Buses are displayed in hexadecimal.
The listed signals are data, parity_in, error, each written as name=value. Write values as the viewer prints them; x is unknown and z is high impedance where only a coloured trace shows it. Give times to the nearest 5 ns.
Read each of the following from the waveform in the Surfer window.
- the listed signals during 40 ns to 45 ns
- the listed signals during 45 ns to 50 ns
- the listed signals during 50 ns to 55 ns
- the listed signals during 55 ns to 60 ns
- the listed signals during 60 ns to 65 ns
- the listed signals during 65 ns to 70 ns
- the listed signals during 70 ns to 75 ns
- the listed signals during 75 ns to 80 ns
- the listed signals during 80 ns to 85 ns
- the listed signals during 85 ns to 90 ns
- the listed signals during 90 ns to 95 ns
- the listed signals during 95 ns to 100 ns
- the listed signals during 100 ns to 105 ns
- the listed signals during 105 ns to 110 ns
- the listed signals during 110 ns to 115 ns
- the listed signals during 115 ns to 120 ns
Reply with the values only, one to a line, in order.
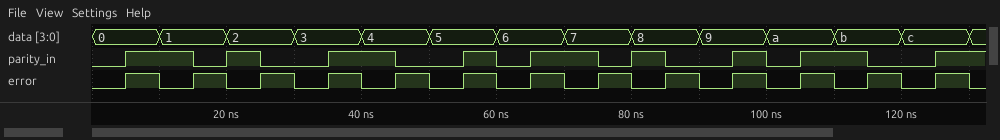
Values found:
data=4, parity_in=1, error=0
data=4, parity_in=0, error=1
data=5, parity_in=0, error=0
data=5, parity_in=1, error=1
data=6, parity_in=0, error=0
data=6, parity_in=1, error=1
data=7, parity_in=1, error=0
data=7, parity_in=0, error=1
data=8, parity_in=1, error=0
data=8, parity_in=0, error=1
data=9, parity_in=0, error=0
data=9, parity_in=1, error=1
data=a, parity_in=0, error=0
data=a, parity_in=1, error=1
data=b, parity_in=1, error=0
data=b, parity_in=0, error=1
